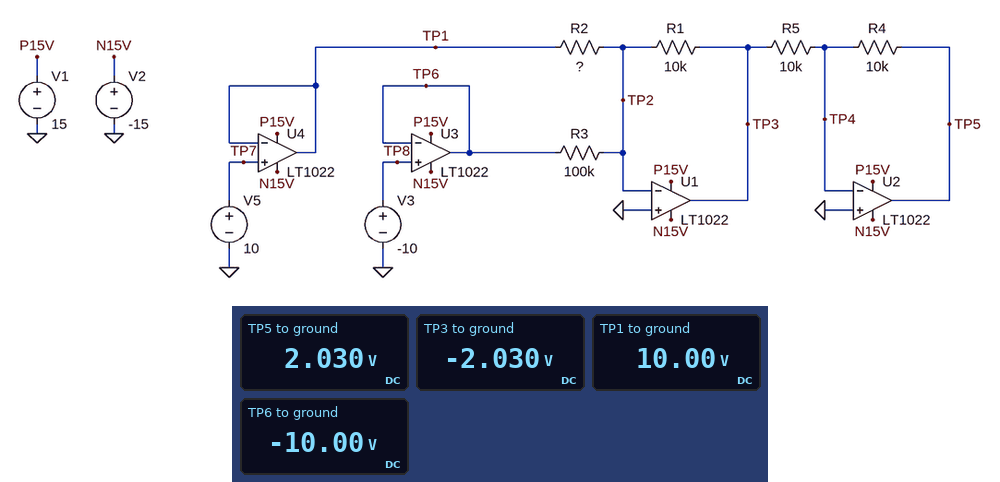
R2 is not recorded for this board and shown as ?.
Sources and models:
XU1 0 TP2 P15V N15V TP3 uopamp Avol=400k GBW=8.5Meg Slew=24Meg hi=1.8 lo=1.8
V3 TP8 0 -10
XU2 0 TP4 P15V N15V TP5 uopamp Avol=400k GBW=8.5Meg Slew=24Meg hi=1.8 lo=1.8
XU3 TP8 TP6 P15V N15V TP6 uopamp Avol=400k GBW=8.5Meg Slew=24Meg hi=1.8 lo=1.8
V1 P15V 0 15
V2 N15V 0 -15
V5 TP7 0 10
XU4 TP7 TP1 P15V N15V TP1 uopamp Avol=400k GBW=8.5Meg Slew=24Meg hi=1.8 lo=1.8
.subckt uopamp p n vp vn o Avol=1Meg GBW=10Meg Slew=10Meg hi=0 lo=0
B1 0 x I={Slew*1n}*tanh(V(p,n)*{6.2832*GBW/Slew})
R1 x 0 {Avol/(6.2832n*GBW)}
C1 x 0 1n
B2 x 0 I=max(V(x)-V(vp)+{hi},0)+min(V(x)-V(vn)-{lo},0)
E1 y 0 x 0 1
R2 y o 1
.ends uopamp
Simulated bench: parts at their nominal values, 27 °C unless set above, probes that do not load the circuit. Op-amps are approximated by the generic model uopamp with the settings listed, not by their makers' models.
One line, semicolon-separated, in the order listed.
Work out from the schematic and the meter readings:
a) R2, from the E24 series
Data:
33 kΩ
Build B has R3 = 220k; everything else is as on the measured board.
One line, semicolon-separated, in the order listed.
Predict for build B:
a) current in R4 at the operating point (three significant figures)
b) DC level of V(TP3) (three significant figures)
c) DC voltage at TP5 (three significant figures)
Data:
258 µA; -2.58 V; 2.58 V
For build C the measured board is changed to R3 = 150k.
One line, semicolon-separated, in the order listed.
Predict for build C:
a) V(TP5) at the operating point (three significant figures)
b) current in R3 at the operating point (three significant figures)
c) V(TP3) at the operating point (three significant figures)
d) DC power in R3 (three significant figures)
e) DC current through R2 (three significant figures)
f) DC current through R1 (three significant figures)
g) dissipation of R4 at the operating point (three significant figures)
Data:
2.36 V; 66.7 µA; -2.36 V; 667 µW; 303 µA; 236 µA; 559 µW
